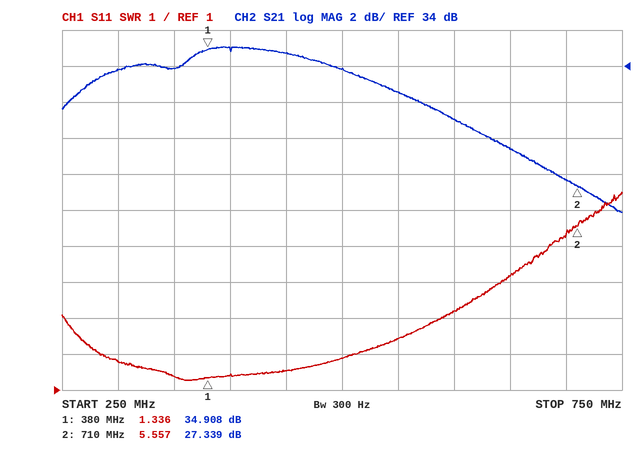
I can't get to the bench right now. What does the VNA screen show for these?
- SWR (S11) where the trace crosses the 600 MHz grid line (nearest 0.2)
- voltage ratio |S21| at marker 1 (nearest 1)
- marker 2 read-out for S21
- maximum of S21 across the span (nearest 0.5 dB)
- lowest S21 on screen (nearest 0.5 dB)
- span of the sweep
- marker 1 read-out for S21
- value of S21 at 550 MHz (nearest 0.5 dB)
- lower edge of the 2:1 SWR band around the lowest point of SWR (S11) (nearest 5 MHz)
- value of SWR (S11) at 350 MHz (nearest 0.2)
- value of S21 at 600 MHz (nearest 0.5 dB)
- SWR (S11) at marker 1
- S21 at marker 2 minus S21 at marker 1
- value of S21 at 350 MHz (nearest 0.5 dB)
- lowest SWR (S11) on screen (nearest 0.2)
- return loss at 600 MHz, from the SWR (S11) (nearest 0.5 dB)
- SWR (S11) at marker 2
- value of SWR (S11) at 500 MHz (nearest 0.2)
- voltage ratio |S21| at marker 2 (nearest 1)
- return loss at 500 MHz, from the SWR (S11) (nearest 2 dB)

3.2
56
27.339 dB
35.0 dB
26.0 dB
500 MHz
34.908 dB
32.5 dB
285 MHz
1.4
31.0 dB
1.336
-7.569 dB
34.0 dB
1.2
5.5 dB
5.557
1.8
23
10 dB
